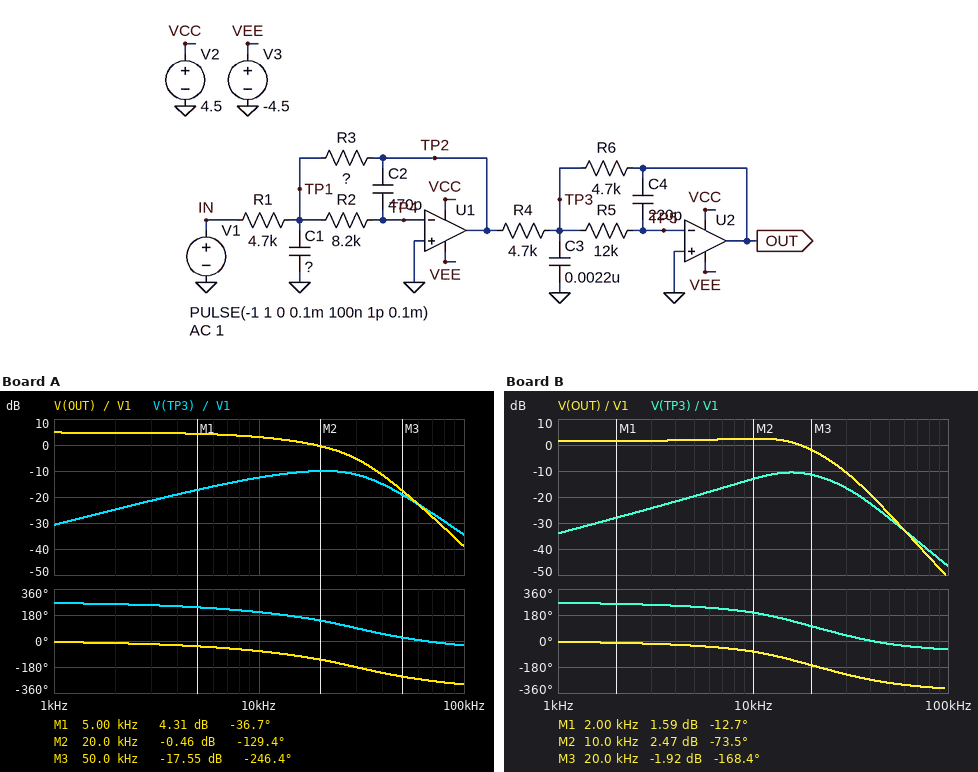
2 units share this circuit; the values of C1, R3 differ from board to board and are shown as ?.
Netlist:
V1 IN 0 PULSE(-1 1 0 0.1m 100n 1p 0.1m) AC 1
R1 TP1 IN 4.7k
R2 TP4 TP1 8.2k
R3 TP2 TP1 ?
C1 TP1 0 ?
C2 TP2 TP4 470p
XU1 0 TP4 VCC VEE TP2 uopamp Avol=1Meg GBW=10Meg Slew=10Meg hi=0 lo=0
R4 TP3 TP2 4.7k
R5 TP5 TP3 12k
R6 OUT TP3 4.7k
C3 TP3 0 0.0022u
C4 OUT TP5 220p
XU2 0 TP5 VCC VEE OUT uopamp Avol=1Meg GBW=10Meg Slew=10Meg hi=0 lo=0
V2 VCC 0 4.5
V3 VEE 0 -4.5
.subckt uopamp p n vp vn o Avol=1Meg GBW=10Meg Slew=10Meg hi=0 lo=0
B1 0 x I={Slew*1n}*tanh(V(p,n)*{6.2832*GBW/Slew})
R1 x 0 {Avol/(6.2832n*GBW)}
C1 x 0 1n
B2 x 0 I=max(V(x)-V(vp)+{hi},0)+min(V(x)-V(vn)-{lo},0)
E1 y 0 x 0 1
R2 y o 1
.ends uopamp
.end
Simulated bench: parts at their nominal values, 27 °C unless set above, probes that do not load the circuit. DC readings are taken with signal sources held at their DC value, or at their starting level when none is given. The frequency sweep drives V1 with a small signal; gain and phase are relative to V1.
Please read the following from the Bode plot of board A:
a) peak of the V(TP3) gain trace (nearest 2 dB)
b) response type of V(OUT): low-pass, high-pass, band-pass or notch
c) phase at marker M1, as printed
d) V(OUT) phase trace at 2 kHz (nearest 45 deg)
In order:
-10 dB
low-pass
-36.7 deg
0 deg
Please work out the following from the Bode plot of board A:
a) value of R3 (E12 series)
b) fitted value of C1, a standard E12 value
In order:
8.2 kΩ
1 nF
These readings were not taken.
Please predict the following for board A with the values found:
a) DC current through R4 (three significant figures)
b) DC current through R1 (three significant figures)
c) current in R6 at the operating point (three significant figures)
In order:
371 µA
213 µA
371 µA
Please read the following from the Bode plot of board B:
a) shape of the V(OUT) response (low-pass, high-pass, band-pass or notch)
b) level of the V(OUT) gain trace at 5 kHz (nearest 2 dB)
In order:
low-pass
2 dB
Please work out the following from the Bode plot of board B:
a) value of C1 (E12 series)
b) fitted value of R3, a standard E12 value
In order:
4.7 nF
5.6 kΩ
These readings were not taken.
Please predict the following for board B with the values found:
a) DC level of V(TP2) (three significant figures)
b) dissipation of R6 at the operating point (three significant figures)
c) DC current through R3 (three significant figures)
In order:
1.19 V
302 µW
213 µA
